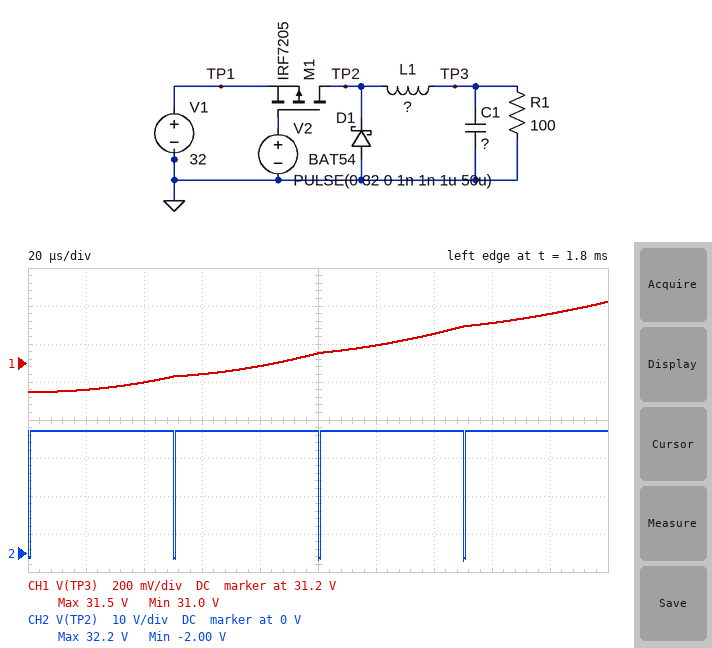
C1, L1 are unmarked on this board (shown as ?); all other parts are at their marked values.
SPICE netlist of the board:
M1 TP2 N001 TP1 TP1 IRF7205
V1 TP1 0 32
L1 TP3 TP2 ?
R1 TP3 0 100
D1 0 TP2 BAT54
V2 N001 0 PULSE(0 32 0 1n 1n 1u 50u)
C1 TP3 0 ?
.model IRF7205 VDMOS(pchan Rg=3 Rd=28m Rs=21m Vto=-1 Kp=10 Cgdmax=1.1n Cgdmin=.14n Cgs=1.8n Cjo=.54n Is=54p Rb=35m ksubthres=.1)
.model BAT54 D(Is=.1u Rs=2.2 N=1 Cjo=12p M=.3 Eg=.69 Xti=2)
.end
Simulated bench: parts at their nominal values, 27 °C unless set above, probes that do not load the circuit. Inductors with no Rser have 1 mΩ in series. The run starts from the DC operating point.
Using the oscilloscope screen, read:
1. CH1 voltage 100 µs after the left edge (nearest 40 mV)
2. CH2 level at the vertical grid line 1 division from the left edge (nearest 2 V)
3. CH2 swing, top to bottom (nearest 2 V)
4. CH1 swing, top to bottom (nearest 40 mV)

31.24 V
32 V
34 V
480 mV
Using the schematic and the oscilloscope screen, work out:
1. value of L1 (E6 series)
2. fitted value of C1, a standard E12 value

330 µH
39 µF
